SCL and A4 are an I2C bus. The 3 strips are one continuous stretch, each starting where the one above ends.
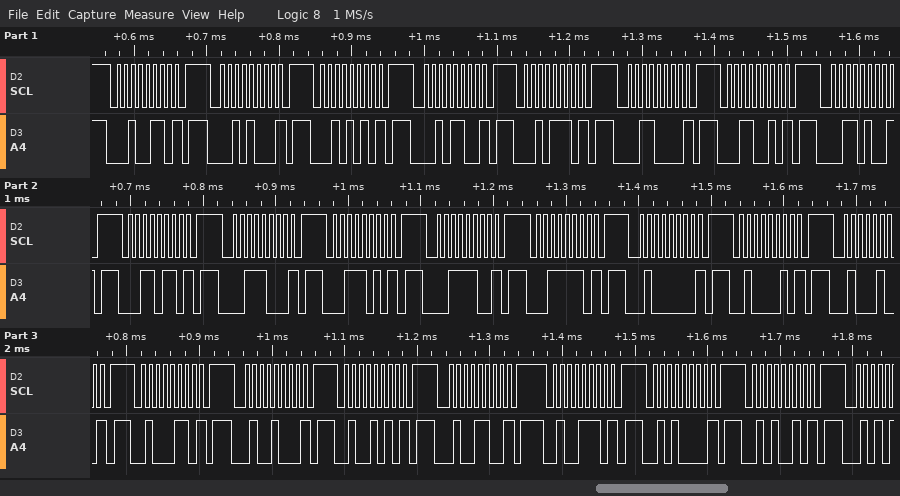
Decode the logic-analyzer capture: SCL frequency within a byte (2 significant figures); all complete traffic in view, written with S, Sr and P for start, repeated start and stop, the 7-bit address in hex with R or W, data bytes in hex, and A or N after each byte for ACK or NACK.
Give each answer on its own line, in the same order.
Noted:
100 kHz
S 13W N P S 14W N P S 15W N P S 16W N P S 17W N P S 18W N P S 19W N P S 1AW N P S 1BW N P S 1CW N P S 1DW N P S 1EW N P S 1FW N P S 20W N P S 21W N P S 22W N P S 23W N P S 24W N P S 25W N P S 26W N P S 27W N P S 28W N P S 29W N P
